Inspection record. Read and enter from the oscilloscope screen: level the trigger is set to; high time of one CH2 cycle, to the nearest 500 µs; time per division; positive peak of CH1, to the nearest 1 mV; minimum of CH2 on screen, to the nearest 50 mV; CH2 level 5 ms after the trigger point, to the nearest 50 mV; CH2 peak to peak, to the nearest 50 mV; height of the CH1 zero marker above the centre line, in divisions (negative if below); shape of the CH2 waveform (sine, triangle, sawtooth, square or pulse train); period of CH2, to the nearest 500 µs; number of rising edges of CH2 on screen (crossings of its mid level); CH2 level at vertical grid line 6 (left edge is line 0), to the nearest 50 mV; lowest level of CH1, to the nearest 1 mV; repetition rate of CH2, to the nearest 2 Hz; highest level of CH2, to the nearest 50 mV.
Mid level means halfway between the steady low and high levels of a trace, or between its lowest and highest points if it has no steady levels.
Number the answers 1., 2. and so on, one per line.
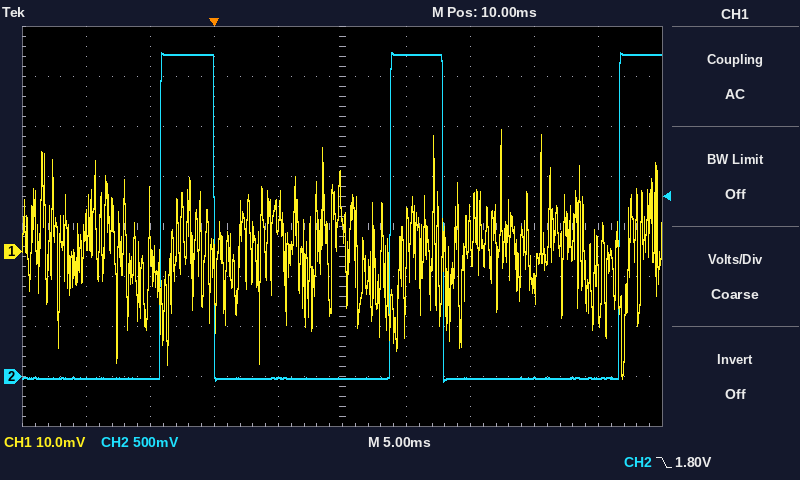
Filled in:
1. 1.80 V
2. 4.0 ms
3. 5 ms
4. 24 mV
5. -50 mV
6. 0 mV
7. 3.30 V
8. -0.5 div
9. pulse train
10. 18.0 ms
11. 3
12. 3.20 V
13. -25 mV
14. 56 Hz
15. 3.25 V
